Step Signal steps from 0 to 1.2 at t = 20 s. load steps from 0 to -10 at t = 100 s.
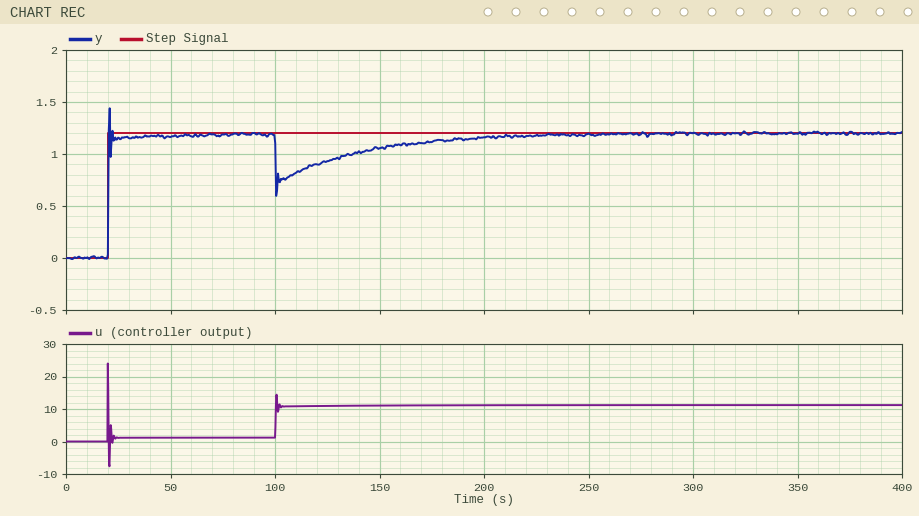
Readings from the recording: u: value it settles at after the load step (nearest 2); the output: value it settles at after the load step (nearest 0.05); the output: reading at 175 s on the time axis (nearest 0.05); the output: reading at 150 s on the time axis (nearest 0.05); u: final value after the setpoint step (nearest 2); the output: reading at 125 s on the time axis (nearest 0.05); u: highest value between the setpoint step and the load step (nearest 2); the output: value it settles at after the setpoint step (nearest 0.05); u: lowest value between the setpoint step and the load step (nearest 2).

12
1.20
1.10
1.05
2
0.95
24
1.20
-8
